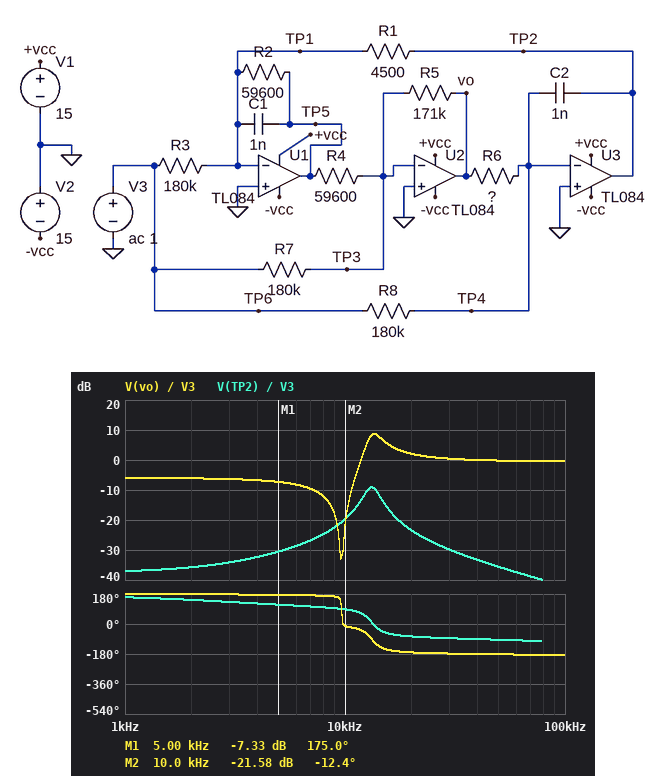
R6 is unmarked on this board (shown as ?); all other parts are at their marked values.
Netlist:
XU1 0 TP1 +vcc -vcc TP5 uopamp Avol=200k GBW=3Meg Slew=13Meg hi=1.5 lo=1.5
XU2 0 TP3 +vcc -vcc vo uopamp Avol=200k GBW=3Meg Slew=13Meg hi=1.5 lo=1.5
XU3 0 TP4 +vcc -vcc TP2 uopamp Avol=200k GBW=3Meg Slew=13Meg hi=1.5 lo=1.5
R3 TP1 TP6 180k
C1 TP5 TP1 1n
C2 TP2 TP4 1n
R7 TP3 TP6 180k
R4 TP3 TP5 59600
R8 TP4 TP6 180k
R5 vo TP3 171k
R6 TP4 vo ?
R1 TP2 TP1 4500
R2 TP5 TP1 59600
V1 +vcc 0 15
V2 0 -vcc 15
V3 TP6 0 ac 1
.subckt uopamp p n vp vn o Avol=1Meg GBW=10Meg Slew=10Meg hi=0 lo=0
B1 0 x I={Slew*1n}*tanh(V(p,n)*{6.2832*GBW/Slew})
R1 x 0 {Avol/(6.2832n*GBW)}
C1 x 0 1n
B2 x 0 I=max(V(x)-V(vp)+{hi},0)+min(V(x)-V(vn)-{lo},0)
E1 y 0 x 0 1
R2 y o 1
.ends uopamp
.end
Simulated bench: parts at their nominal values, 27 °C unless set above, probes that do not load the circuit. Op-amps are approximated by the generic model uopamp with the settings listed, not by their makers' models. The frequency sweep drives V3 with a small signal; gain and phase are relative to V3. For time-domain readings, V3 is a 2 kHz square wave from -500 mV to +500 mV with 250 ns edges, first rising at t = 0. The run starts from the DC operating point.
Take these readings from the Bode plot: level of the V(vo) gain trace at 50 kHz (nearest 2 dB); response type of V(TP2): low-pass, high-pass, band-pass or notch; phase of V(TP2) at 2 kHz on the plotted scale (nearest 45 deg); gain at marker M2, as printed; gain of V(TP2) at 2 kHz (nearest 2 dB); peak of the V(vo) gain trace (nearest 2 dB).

0 dB
band-pass
135 deg
-21.58 dB
-36 dB
8 dB
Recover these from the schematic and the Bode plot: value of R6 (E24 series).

91 kΩ
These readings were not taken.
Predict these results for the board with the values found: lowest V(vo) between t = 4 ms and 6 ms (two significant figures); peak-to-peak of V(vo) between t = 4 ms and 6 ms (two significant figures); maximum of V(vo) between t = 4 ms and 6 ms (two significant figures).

-710 mV
1.4 V
710 mV
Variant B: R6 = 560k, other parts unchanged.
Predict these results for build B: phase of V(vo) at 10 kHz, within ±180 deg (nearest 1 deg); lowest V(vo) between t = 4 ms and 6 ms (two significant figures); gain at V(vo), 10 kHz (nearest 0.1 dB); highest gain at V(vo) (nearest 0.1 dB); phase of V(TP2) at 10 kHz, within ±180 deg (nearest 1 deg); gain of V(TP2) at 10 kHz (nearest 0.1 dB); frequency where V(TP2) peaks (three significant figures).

-156 deg
-2.6 V
-21.4 dB
13.9 dB
89 deg
-21.3 dB
5.23 kHz
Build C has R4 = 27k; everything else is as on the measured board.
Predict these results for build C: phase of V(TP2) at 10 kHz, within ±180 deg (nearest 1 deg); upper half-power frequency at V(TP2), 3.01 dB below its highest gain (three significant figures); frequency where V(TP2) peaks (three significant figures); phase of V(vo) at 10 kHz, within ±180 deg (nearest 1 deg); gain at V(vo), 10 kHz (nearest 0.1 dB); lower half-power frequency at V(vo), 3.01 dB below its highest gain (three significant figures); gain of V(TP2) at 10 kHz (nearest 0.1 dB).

129 deg
20.3 kHz
19.6 kHz
158 deg
-8.7 dB
19.1 kHz
-28.6 dB
